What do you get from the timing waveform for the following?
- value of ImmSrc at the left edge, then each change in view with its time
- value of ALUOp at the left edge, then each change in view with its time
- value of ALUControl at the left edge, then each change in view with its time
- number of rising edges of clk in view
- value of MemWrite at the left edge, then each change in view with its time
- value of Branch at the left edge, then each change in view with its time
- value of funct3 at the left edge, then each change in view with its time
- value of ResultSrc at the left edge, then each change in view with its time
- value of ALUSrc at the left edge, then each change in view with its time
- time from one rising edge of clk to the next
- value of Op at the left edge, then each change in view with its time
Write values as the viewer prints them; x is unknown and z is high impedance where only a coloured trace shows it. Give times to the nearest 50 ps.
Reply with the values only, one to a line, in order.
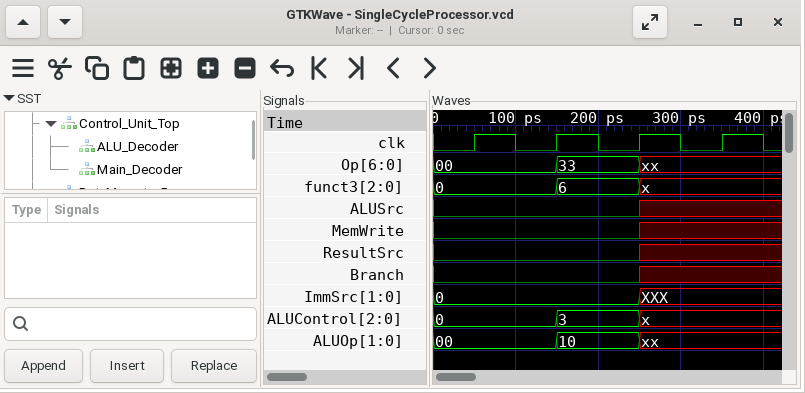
0, XXX at 250 ps
00, 10 at 150 ps, xx at 250 ps
0, 3 at 150 ps, x at 250 ps
4
0, x at 250 ps
0, x at 250 ps
0, 6 at 150 ps, x at 250 ps
0, x at 250 ps
0, x at 250 ps
100 ps
00, 33 at 150 ps, xx at 250 ps
